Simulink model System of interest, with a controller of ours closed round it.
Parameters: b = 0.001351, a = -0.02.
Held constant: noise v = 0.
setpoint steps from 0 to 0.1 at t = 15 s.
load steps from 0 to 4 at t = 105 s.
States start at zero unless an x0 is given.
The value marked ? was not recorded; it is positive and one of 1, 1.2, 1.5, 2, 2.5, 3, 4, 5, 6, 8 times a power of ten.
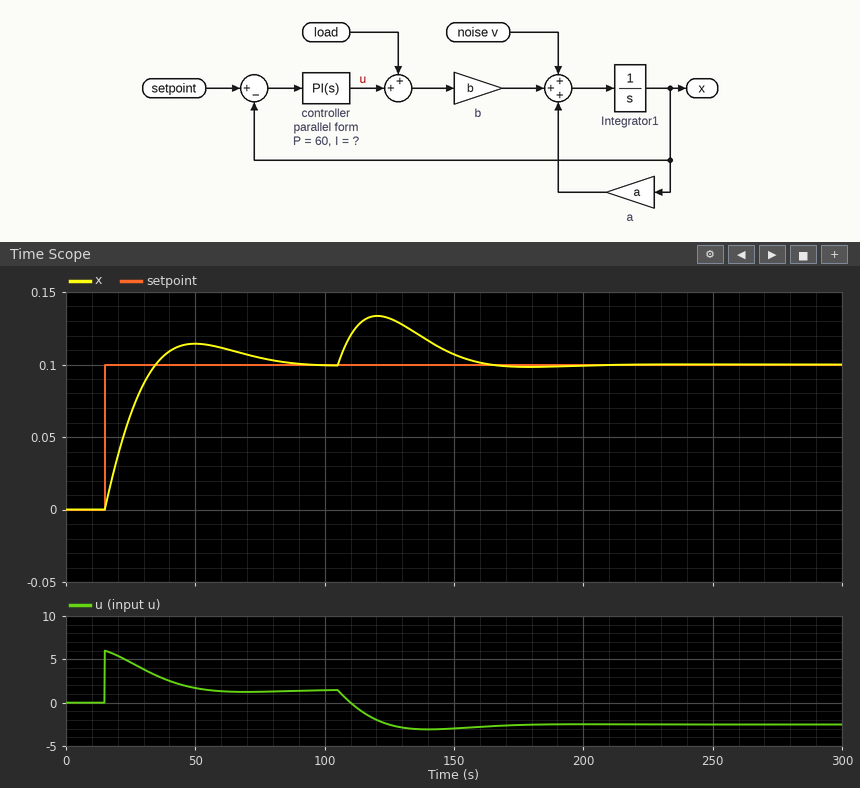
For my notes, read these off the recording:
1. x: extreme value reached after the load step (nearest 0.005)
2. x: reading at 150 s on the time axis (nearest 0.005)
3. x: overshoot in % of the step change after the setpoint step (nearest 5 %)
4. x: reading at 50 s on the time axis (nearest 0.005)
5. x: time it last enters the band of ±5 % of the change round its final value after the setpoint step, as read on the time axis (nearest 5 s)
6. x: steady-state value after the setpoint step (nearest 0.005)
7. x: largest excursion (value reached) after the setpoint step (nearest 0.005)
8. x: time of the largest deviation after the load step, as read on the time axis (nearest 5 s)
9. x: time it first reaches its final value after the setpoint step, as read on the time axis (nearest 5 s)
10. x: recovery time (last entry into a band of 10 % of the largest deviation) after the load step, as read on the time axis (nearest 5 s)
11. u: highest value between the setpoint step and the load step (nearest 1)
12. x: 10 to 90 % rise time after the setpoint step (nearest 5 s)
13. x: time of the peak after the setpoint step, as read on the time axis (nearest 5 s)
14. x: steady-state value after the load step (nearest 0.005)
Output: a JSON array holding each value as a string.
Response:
["0.135", "0.105", "15 %", "0.115", "75 s", "0.100", "0.115", "120 s", "35 s", "155 s", "6", "15 s", "50 s", "0.100"]
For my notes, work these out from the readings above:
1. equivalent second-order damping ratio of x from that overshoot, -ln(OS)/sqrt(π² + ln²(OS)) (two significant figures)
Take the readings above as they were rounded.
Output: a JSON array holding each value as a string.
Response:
["0.52"]
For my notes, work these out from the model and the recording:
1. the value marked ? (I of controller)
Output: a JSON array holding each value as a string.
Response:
["4"]
